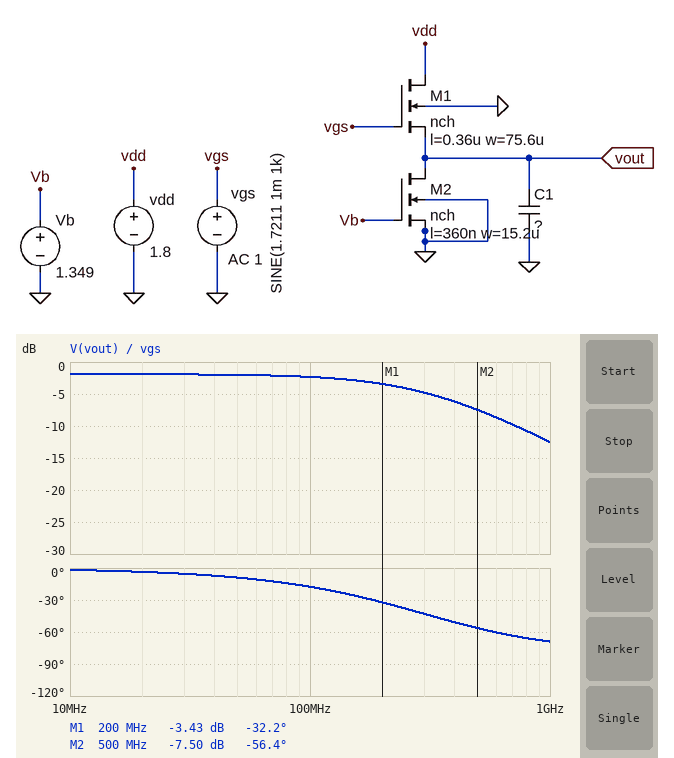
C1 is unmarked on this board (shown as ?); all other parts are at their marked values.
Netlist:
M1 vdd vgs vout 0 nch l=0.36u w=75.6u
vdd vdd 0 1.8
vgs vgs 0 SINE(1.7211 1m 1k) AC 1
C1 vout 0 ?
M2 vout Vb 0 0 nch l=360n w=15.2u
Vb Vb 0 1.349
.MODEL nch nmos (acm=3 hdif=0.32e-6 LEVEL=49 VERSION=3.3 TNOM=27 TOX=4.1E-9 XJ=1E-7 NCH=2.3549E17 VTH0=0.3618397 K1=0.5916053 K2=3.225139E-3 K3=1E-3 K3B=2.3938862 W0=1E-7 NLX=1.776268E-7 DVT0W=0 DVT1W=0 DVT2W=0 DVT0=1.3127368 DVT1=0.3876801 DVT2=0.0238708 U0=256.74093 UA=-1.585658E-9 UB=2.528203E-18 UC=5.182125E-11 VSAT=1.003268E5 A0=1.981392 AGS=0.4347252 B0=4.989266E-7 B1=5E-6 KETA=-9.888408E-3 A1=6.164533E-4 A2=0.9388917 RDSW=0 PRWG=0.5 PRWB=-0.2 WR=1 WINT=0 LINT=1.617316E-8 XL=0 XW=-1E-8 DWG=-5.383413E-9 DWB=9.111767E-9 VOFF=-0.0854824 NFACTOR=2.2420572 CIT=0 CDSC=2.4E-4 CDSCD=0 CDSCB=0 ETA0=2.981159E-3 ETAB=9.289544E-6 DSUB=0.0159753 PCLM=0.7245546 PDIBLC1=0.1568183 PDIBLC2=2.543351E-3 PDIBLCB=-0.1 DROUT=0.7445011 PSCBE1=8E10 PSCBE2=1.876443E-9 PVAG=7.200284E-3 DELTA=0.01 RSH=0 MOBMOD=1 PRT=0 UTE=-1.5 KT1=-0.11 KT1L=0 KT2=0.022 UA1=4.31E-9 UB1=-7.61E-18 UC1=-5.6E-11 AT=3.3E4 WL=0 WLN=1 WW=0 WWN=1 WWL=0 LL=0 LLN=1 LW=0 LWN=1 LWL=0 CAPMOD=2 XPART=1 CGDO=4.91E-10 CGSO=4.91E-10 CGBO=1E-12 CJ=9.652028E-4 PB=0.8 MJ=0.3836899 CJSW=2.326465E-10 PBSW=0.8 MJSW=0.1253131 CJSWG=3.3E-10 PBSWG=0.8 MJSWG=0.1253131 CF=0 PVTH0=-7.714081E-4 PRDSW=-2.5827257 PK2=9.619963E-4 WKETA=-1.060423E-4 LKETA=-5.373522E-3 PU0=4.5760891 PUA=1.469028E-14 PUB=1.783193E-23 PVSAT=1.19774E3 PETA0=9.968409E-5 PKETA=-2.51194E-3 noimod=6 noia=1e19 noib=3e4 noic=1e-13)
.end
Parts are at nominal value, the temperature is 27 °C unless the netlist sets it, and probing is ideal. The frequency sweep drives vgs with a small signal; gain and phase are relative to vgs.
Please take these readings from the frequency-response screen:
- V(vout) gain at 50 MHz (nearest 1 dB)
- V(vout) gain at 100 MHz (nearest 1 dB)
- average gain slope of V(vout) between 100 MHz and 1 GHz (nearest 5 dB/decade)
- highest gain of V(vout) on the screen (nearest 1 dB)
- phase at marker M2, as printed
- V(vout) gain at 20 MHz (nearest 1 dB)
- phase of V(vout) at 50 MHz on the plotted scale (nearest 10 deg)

-2 dB
-2 dB
-10 dB/decade
-2 dB
-56.4 deg
-2 dB
-10 deg
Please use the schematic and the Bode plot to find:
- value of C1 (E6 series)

10 pF
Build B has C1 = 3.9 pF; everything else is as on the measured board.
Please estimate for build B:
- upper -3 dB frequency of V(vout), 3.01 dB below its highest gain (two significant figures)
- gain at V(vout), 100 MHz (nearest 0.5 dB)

760 MHz
-2.0 dB
